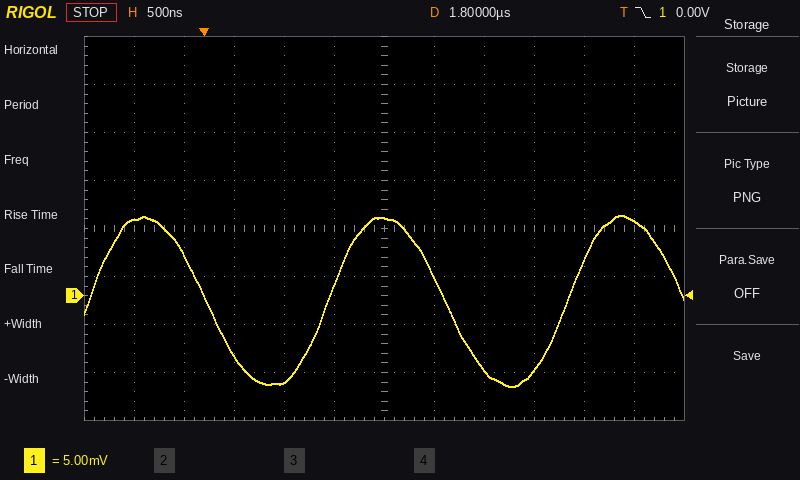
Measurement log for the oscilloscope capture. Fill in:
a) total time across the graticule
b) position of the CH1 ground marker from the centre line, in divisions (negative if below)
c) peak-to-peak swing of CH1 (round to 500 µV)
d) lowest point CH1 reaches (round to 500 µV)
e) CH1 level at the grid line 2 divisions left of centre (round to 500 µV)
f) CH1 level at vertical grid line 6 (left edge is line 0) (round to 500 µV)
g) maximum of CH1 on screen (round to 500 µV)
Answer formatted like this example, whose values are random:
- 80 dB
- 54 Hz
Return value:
- 6 µs
- -1.4 div
- 18.0 mV
- -9.5 mV
- -9.0 mV
- 8.0 mV
- 8.5 mV
